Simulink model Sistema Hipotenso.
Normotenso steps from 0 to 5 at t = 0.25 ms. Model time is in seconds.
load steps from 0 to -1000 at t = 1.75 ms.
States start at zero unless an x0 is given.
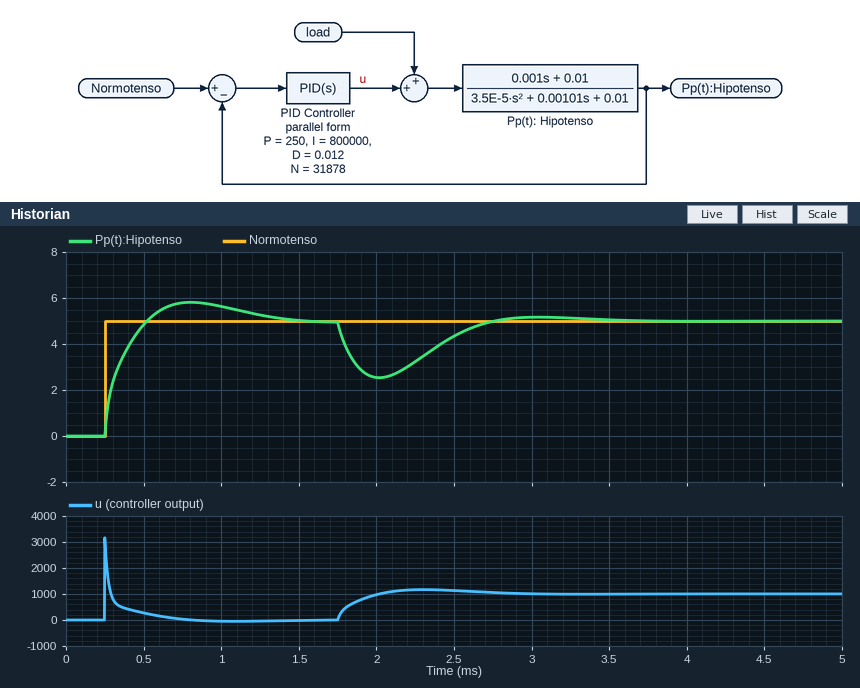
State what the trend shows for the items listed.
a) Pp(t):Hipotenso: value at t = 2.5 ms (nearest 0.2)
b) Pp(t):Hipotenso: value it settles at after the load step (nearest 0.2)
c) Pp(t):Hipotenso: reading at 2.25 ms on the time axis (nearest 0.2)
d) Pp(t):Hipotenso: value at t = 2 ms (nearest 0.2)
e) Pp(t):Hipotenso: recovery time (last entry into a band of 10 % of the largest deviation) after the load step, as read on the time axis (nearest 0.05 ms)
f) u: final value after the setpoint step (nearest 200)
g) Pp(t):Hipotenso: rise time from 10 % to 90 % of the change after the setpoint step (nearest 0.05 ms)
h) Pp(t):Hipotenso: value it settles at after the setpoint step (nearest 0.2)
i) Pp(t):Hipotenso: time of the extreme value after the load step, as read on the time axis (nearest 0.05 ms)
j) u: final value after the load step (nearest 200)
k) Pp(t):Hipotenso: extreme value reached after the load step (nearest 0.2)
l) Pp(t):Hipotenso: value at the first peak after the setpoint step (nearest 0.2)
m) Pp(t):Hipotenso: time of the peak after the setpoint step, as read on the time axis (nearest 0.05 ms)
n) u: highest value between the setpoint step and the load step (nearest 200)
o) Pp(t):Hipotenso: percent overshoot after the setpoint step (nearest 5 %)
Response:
4.4
5.0
3.2
2.6
2.65 ms
0
0.20 ms
5.0
2.00 ms
1000
2.6
5.8
0.80 ms
3200
15 %
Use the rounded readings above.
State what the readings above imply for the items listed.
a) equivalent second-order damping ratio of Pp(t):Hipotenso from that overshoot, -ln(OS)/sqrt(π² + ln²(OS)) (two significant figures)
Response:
0.52
